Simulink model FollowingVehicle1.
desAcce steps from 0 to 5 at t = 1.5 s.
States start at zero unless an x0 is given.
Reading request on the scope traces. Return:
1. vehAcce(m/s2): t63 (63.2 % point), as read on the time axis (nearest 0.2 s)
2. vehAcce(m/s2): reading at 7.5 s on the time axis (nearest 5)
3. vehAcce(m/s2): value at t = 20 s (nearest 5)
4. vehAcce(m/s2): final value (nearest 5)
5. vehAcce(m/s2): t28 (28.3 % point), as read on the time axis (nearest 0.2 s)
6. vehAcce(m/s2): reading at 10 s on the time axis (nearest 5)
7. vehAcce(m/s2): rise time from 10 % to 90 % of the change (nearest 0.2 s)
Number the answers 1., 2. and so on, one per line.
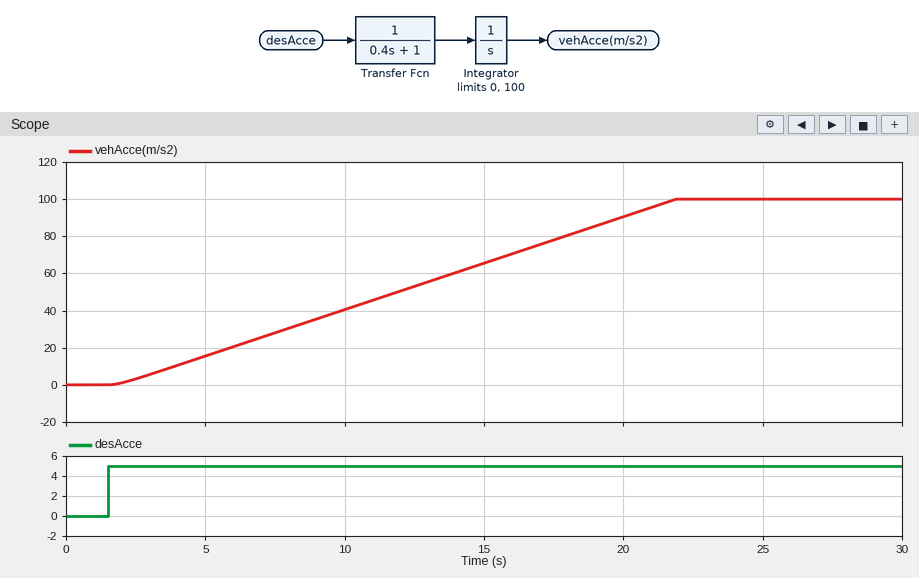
1. 14.6 s
2. 30
3. 90
4. 100
5. 7.6 s
6. 40
7. 16.0 s
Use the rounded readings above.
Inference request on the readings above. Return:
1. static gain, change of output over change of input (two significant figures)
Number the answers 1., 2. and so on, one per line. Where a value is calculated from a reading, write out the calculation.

1. (100 - 0) / (5 - 0) = 20
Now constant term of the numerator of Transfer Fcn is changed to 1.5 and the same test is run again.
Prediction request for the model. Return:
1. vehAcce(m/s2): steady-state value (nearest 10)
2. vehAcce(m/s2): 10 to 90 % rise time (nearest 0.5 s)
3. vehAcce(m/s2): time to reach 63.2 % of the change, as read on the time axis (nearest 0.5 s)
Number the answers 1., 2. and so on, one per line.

1. 100
2. 10.5 s
3. 10.5 s
